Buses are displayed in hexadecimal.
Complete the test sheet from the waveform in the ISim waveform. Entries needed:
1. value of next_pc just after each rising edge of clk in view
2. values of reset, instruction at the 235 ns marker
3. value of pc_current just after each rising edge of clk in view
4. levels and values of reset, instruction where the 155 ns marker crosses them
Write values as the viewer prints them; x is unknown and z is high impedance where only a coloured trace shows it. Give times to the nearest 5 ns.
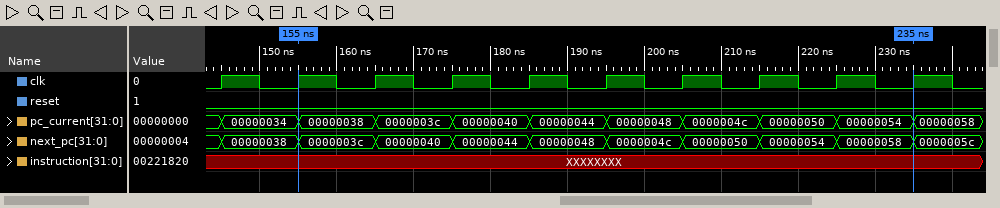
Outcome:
00000038, 0000003c, 00000040, 00000044, 00000048, 0000004c, 00000050, 00000054, 00000058, 0000005c
reset=0, instruction=XXXXXXXX
00000034, 00000038, 0000003c, 00000040, 00000044, 00000048, 0000004c, 00000050, 00000054, 00000058
reset=0, instruction=XXXXXXXX
